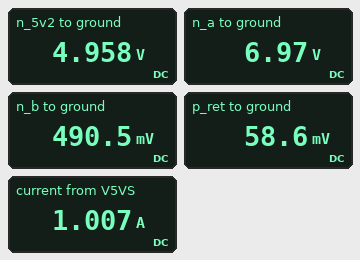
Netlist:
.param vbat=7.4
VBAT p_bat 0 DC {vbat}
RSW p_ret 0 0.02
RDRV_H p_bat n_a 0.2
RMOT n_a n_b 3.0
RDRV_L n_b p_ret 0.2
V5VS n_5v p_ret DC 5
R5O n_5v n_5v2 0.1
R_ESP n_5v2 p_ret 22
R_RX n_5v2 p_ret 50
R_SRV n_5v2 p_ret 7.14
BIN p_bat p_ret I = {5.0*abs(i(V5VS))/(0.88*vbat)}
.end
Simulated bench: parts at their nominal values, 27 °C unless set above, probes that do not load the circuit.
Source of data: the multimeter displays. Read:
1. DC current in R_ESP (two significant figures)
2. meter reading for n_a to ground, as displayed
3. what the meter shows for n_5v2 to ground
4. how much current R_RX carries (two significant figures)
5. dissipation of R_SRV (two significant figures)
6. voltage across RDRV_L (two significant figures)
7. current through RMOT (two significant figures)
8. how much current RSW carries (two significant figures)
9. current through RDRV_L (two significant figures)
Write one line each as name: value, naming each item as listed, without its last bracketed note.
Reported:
DC current in R_ESP: 220 mA
meter reading for n_a to ground, as displayed: 6.97 V
what the meter shows for n_5v2 to ground: 4.958 V
how much current R_RX carries: 98 mA
dissipation of R_SRV: 3.4 W
voltage across RDRV_L: 430 mV
current through RMOT: 2.2 A
how much current RSW carries: 2.9 A
current through RDRV_L: 2.2 A
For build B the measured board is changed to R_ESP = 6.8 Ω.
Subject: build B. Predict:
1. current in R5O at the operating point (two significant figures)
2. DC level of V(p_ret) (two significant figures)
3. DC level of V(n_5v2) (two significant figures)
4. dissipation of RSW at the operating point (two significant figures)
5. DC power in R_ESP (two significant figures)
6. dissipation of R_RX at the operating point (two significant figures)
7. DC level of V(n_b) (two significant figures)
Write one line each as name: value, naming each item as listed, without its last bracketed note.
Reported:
current in R5O at the operating point: 1.5 A
DC level of V(p_ret): 66 mV
DC level of V(n_5v2): 4.9 V
dissipation of RSW at the operating point: 220 mW
DC power in R_ESP: 3.5 W
dissipation of R_RX at the operating point: 470 mW
DC level of V(n_b): 500 mV
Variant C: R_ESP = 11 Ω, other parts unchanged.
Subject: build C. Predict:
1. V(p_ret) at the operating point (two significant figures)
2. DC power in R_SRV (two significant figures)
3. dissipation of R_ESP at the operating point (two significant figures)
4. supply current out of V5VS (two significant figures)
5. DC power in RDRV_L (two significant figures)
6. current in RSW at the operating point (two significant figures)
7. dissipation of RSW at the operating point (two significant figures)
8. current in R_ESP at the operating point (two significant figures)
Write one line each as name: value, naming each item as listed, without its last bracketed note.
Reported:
V(p_ret) at the operating point: 62 mV
DC power in R_SRV: 3.3 W
dissipation of R_ESP at the operating point: 2.2 W
supply current out of V5VS: 1.2 A
DC power in RDRV_L: 930 mW
current in RSW at the operating point: 3.1 A
dissipation of RSW at the operating point: 190 mW
current in R_ESP at the operating point: 440 mA
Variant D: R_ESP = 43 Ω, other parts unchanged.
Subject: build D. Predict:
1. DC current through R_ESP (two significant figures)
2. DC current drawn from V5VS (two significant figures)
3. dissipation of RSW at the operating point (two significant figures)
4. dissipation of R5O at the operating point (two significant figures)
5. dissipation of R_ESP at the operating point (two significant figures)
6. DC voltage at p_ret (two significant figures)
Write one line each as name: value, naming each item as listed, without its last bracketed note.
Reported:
DC current through R_ESP: 110 mA
DC current drawn from V5VS: 900 mA
dissipation of RSW at the operating point: 160 mW
dissipation of R5O at the operating point: 81 mW
dissipation of R_ESP at the operating point: 560 mW
DC voltage at p_ret: 57 mV
